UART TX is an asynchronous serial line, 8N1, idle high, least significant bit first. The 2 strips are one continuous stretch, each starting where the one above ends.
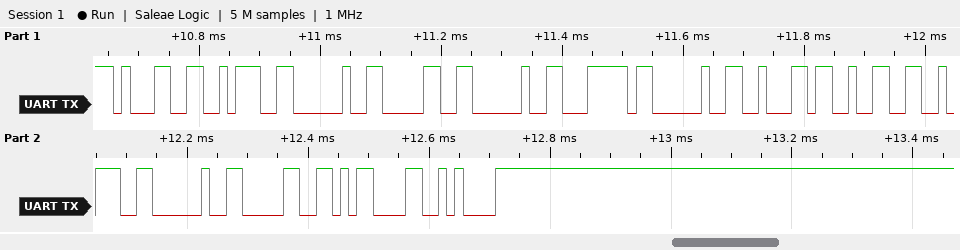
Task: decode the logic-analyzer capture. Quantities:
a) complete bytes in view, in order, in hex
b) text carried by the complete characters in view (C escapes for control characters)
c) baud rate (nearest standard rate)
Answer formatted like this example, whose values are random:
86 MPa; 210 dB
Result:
31 3A 20 30 20 7C 20 62 32 3A 20 30 0D 0A; "1: 0 | b2: 0\r\n"; 74880 baud
